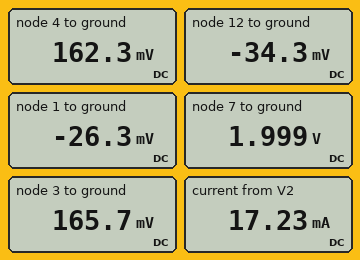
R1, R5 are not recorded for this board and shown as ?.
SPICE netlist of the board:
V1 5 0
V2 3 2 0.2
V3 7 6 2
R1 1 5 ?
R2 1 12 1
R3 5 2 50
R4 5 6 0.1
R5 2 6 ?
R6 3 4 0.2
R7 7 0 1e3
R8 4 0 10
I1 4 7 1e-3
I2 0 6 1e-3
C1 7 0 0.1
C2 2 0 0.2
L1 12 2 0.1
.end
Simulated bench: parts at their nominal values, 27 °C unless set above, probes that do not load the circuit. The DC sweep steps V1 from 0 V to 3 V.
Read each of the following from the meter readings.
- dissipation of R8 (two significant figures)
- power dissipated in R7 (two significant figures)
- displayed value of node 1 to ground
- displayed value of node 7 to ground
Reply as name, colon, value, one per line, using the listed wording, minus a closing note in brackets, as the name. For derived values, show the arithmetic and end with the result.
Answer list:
dissipation of R8: (162.3 mV)^2 / 10 Ω = 2.6 mW
power dissipated in R7: (1.999 V)^2 / 1 kΩ = 4.0 mW
displayed value of node 1 to ground: -26.3 mV
displayed value of node 7 to ground: 1.999 V
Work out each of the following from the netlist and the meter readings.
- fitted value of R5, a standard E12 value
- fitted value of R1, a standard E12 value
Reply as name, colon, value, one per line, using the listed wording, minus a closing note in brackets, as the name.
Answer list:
fitted value of R5, a standard E12 value: 3.9 Ω
fitted value of R1, a standard E12 value: 3.3 Ω
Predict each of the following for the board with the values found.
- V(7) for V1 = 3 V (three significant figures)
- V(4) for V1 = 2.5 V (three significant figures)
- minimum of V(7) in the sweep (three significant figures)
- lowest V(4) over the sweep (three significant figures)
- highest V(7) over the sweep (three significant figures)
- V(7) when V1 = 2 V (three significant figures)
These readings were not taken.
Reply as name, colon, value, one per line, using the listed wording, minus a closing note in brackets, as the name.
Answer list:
V(7) for V1 = 3 V: 4.99 V
V(4) for V1 = 2.5 V: 2.21 V
minimum of V(7) in the sweep: 2.00 V
lowest V(4) over the sweep: 162 mV
highest V(7) over the sweep: 4.99 V
V(7) when V1 = 2 V: 3.99 V
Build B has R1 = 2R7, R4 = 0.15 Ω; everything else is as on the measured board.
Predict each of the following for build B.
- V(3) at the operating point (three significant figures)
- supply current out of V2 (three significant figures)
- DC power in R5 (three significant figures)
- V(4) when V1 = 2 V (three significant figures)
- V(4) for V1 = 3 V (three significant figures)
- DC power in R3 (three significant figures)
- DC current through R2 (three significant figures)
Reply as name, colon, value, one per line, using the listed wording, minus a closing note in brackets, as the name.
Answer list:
V(3) at the operating point: 168 mV
supply current out of V2: 17.4 mA
DC power in R5: 250 µW
V(4) when V1 = 2 V: 1.82 V
V(4) for V1 = 3 V: 2.65 V
DC power in R3: 21.0 µW
DC current through R2: 8.76 mA
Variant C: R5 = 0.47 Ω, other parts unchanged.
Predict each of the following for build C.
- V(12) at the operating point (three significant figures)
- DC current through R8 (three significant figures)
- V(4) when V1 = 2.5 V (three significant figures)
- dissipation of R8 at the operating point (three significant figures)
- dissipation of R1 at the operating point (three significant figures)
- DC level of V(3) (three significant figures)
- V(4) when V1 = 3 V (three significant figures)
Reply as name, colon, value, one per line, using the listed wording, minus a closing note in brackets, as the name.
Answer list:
V(12) at the operating point: -9.78 mV
DC current through R8: 18.6 mA
V(4) when V1 = 2.5 V: 2.52 V
dissipation of R8 at the operating point: 3.47 mW
dissipation of R1 at the operating point: 17.1 µW
DC level of V(3): 190 mV
V(4) when V1 = 3 V: 2.99 V
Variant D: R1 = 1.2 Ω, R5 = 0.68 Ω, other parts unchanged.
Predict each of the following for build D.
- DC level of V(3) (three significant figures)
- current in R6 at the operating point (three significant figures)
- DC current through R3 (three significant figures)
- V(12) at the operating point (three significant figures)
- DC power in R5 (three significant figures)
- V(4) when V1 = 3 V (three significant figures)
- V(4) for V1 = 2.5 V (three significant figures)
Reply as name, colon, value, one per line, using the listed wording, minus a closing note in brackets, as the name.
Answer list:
DC level of V(3): 189 mV
current in R6 at the operating point: 19.5 mA
DC current through R3: 222 µA
V(12) at the operating point: -11.1 mV
DC power in R5: 138 µW
V(4) when V1 = 3 V: 2.97 V
V(4) for V1 = 2.5 V: 2.51 V
